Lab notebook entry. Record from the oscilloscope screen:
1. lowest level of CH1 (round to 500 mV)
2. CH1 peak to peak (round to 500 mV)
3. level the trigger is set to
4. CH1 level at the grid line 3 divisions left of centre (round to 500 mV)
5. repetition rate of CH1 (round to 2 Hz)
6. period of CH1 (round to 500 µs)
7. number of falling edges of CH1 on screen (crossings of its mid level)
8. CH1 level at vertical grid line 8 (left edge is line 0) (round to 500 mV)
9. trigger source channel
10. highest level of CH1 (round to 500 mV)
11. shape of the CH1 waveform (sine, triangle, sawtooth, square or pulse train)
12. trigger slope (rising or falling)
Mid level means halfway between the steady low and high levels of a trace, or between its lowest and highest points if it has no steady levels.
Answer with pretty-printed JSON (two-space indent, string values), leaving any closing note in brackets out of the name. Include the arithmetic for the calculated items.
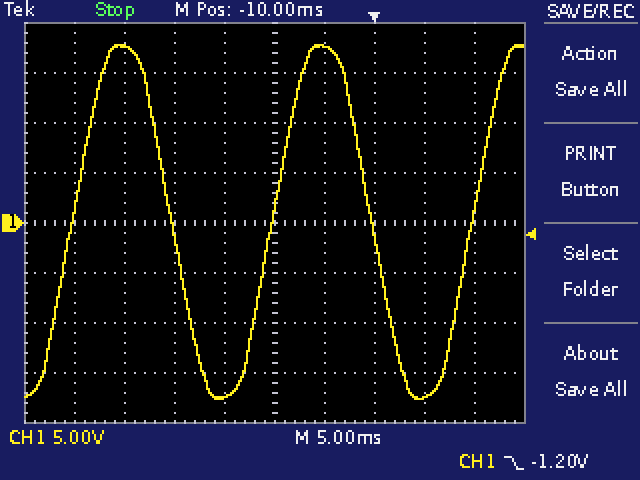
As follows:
{
  "lowest level of CH1": "-17.5 V",
  "CH1 peak to peak": "18.0 V − (-17.5 V) = 35.5 V",
  "level the trigger is set to": "-1.20 V",
  "CH1 level at the grid line 3 divisions left of centre": "17.5 V",
  "repetition rate of CH1": "1 / 20.0 ms ≈ 50 Hz",
  "period of CH1": "20.0 ms",
  "number of falling edges of CH1 on screen": "2",
  "CH1 level at vertical grid line 8 (left edge is line 0)": "-17.5 V",
  "trigger source channel": "CH1",
  "highest level of CH1": "18.0 V",
  "shape of the CH1 waveform": "sine",
  "trigger slope": "falling"
}
